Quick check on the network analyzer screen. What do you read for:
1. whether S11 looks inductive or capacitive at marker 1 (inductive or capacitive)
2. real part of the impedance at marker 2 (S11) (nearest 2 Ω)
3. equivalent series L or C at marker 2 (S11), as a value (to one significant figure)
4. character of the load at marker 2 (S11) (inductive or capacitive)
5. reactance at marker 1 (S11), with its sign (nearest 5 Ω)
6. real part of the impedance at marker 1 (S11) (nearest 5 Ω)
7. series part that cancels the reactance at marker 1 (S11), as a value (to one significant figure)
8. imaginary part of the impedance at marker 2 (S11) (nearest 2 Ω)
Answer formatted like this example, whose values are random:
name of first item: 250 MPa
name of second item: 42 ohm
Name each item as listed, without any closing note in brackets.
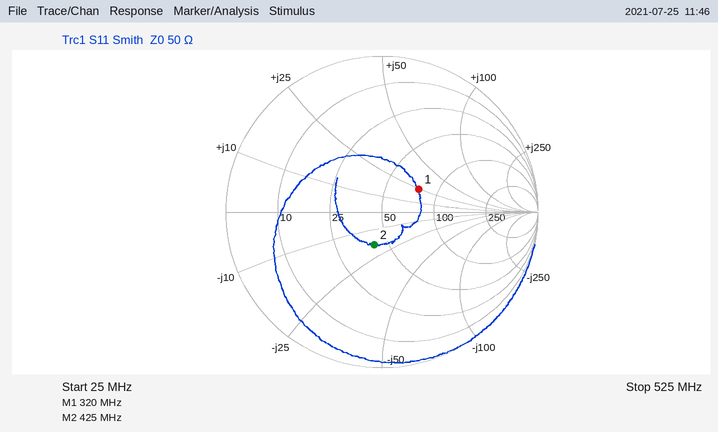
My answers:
whether S11 looks inductive or capacitive at marker 1: inductive
real part of the impedance at marker 2 (S11): 42 Ω
equivalent series L or C at marker 2 (S11), as a value: 20 pF
character of the load at marker 2 (S11): capacitive
reactance at marker 1 (S11), with its sign: +25 Ω
real part of the impedance at marker 1 (S11): 75 Ω
series part that cancels the reactance at marker 1 (S11), as a value: 20 pF
imaginary part of the impedance at marker 2 (S11): -18 Ω
